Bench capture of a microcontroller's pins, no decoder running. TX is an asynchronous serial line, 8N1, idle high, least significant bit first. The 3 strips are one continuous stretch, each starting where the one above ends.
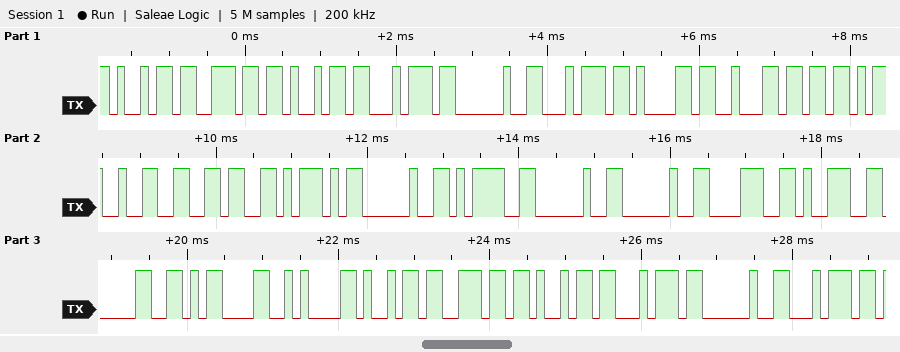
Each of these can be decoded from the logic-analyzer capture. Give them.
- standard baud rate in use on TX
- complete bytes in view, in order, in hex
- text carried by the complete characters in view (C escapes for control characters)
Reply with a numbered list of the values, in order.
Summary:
1. 9600 baud
2. 0x69 0x6E 0x69 0x74 0x20 0x74 0x61 0x62 0x5B 0x32 0x36 0x5D 0x20 0x3D 0x20 0x20 0x38 0x39 0x30 0x0D 0x0A 0x69 0x6E 0x69 0x74 0x20 0x74
3. "init tab[26] =  890\r\ninit t"
